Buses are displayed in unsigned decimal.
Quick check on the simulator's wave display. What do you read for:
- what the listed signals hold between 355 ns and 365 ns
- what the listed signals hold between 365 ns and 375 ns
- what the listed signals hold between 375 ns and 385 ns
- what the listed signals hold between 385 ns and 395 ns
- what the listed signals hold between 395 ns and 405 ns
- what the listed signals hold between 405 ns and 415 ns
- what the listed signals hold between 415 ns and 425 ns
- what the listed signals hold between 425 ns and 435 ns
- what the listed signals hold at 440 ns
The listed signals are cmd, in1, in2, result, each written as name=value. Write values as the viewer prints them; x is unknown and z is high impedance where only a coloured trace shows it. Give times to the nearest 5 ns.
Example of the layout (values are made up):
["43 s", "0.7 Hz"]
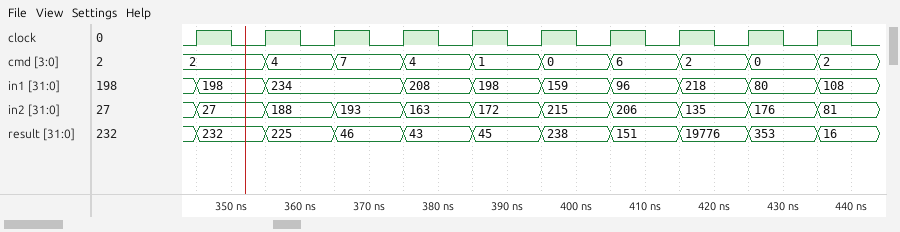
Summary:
["cmd=4, in1=234, in2=188, result=225", "cmd=7, in1=234, in2=193, result=46", "cmd=4, in1=208, in2=163, result=43", "cmd=1, in1=198, in2=172, result=45", "cmd=0, in1=159, in2=215, result=238", "cmd=6, in1=96, in2=206, result=151", "cmd=2, in1=218, in2=135, result=19776", "cmd=0, in1=80, in2=176, result=353", "cmd=2, in1=108, in2=81, result=16"]
